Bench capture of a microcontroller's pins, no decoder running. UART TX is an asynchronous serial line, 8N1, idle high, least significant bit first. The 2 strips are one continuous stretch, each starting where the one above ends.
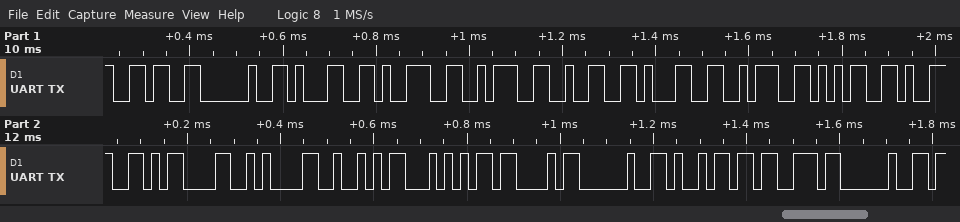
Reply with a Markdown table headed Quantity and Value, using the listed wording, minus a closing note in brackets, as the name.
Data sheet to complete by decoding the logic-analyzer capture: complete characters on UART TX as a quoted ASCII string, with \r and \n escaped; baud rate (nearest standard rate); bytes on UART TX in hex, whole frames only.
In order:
| Quantity | Value |
|---|---|
| complete characters on UART TX as a quoted ASCII string, with \r and \n escaped | "6 19:21:59\r\nRTC is " |
| baud rate | 57600 baud |
| bytes on UART TX in hex, whole frames only | 36 20 31 39 3A 32 31 3A 35 39 0D 0A 52 54 43 20 69 73 20 |
